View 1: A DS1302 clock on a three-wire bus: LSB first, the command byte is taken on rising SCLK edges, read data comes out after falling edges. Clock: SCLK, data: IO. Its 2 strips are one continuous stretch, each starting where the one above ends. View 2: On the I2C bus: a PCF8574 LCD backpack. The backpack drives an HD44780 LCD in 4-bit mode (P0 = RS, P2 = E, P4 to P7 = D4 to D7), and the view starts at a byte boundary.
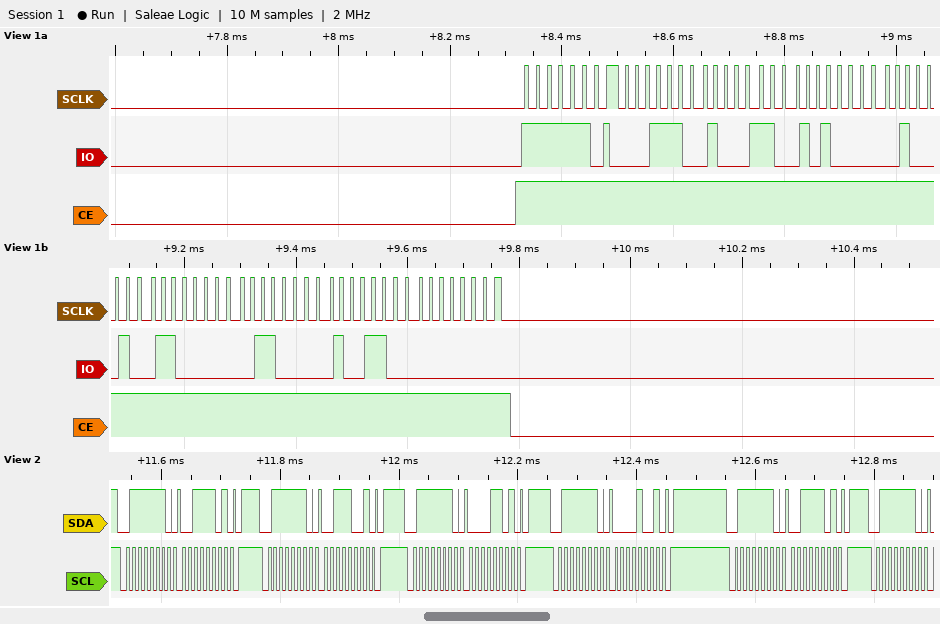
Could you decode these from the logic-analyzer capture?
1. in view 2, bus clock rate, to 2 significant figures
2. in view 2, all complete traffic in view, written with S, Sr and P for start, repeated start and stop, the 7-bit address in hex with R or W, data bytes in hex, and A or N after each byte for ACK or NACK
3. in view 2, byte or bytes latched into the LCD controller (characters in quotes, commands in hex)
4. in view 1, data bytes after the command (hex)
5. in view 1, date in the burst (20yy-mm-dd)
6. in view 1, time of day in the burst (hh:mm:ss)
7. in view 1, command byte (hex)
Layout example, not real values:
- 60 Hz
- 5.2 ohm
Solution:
- 100 kHz
- S 3FW A 3D A P S 3FW A 39 A P S 3FW A 0D A P S 3FW A 09 A P S 3FW A 3D A P S 3FW A
- '0'
- 38 31 05 22 03 06 19 00
- 2019-03-22
- 05:31:38
- 0xBF
